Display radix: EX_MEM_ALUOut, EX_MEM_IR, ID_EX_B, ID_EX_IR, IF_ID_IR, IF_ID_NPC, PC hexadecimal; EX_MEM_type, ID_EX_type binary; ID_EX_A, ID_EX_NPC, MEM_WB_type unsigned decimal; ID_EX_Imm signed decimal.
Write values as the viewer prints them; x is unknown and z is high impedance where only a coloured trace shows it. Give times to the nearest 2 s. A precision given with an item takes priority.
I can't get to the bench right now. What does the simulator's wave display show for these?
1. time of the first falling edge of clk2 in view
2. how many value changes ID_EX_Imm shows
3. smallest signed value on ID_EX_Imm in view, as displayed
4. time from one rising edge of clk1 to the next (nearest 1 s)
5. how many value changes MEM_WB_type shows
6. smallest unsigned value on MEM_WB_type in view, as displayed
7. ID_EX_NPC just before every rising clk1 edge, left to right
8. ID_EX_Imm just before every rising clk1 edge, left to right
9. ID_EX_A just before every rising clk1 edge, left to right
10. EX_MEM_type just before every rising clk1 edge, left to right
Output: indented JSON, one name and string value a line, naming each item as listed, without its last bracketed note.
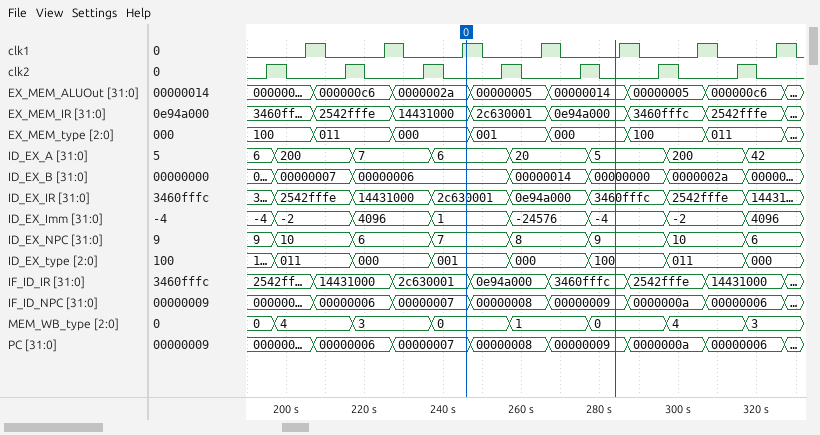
{
  "time of the first falling edge of clk2 in view": "200 s",
  "how many value changes ID_EX_Imm shows": "7",
  "smallest signed value on ID_EX_Imm in view, as displayed": "-24576",
  "time from one rising edge of clk1 to the next": "20 s",
  "how many value changes MEM_WB_type shows": "7",
  "smallest unsigned value on MEM_WB_type in view, as displayed": "0",
  "ID_EX_NPC just before every rising clk1 edge, left to right": "10, 6, 7, 8, 9, 10, 6",
  "ID_EX_Imm just before every rising clk1 edge, left to right": "-2, 4096, 1, -24576, -4, -2, 4096",
  "ID_EX_A just before every rising clk1 edge, left to right": "200, 7, 6, 20, 5, 200, 42",
  "EX_MEM_type just before every rising clk1 edge, left to right": "100, 011, 000, 001, 000, 100, 011"
}
